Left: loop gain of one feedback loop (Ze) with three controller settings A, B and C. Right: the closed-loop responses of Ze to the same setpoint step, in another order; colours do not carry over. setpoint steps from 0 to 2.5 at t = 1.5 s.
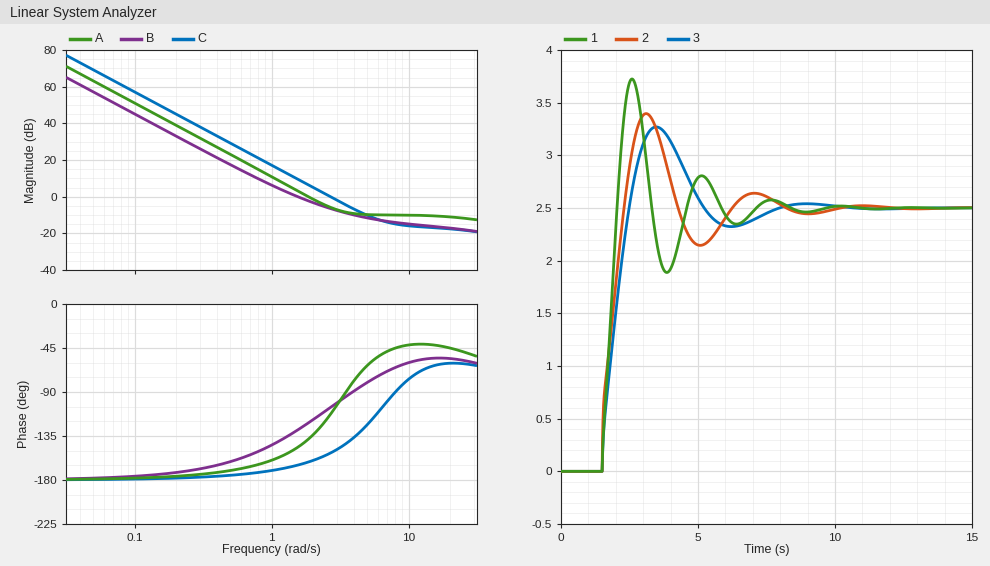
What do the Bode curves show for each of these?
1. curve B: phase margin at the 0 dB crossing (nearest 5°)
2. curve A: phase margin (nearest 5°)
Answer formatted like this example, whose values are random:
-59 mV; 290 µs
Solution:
50°; 40°
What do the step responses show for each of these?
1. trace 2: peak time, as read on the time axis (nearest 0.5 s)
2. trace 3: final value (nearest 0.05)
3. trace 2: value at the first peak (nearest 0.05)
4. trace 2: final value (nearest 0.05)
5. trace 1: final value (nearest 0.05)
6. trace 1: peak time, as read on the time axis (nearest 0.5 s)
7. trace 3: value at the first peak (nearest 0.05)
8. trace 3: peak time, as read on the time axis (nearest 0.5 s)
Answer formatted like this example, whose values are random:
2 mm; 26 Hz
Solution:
3.0 s; 2.50; 3.40; 2.50; 2.50; 2.5 s; 3.25; 3.5 s
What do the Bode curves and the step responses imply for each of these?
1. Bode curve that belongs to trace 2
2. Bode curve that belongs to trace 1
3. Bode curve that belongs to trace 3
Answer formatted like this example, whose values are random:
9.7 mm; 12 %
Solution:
A; C; B
